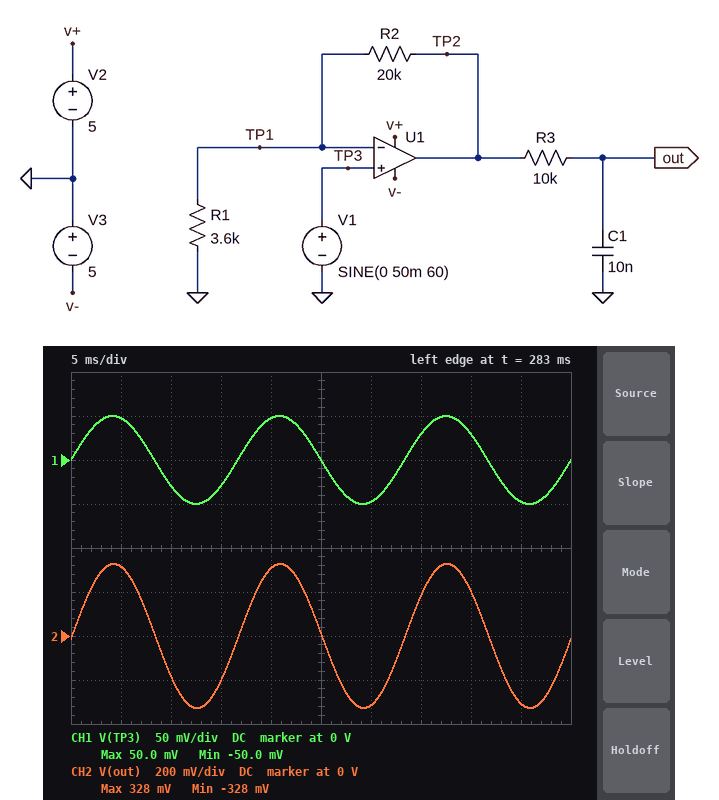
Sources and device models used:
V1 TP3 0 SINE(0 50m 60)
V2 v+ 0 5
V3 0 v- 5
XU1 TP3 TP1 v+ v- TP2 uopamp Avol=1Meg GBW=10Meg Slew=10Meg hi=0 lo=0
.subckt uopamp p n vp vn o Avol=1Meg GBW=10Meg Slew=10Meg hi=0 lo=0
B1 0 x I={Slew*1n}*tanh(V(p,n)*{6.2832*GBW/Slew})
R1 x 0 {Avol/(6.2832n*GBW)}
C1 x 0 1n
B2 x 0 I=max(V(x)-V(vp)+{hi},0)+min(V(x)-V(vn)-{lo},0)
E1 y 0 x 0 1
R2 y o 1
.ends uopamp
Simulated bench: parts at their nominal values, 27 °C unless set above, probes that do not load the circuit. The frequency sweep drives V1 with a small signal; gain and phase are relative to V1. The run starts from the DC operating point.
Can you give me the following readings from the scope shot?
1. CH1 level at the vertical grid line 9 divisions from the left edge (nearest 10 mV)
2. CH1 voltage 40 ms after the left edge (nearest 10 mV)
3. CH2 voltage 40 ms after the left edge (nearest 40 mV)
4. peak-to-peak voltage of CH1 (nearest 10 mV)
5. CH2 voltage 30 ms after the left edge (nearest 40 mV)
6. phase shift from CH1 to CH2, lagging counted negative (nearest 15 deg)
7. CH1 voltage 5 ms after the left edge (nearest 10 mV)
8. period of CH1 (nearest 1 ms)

-50 mV
30 mV
200 mV
100 mV
-320 mV
0 deg
50 mV
17 ms
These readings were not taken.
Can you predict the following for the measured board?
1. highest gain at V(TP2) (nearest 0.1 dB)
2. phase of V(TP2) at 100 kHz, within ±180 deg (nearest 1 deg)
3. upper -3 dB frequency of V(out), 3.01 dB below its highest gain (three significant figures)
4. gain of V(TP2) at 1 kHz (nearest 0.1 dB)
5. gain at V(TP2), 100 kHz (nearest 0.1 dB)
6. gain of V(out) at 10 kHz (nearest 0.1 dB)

16.3 dB
-4 deg
1.59 kHz
16.3 dB
16.3 dB
0.3 dB
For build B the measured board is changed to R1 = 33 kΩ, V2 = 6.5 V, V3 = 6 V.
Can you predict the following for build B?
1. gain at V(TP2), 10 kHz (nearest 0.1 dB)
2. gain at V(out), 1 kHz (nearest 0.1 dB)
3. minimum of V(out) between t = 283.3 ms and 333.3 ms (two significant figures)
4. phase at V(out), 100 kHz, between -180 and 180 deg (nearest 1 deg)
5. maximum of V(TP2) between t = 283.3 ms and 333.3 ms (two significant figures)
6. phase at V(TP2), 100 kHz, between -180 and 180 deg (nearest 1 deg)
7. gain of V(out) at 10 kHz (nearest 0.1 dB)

4.1 dB
2.7 dB
-80 mV
-90 deg
80 mV
-1 deg
-12.0 dB
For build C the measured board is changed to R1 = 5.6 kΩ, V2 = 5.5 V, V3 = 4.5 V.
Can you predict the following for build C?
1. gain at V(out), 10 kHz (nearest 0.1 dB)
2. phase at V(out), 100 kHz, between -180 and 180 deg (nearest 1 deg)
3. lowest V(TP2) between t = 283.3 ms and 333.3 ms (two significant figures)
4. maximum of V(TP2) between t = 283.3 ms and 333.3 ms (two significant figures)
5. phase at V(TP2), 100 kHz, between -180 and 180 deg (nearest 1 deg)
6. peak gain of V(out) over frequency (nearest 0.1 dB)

-2.9 dB
-92 deg
-230 mV
230 mV
-3 deg
13.2 dB
